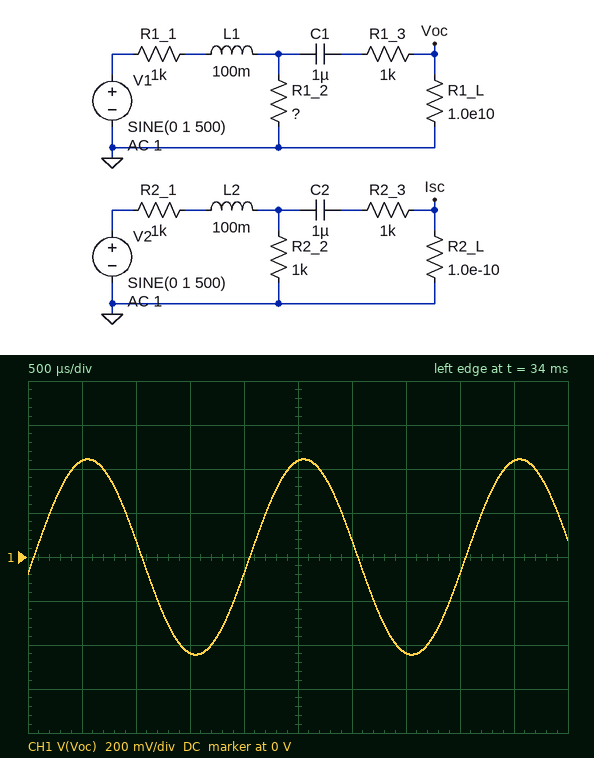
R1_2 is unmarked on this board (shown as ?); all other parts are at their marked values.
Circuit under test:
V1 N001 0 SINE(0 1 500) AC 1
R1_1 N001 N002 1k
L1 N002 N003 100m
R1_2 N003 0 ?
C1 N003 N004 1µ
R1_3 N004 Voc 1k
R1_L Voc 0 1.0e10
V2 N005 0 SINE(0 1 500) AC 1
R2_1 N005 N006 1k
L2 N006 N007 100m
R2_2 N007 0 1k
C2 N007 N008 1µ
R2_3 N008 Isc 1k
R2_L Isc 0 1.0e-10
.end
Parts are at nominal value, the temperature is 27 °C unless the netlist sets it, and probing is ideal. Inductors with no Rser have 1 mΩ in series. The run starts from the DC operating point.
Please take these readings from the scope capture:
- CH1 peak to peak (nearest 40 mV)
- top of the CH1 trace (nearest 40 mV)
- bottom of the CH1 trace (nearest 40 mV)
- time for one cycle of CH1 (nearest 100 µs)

880 mV
440 mV
-440 mV
2.0 ms
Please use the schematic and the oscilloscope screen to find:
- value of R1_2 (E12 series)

820 Ω
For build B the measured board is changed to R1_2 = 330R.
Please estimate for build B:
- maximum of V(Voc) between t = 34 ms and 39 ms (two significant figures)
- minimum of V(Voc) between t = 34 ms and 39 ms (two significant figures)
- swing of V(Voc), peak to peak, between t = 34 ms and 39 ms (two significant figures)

240 mV
-240 mV
480 mV
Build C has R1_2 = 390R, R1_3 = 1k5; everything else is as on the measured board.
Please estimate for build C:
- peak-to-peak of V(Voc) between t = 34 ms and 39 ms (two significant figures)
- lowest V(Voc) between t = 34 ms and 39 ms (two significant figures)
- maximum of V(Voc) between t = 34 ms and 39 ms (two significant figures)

550 mV
-270 mV
270 mV
